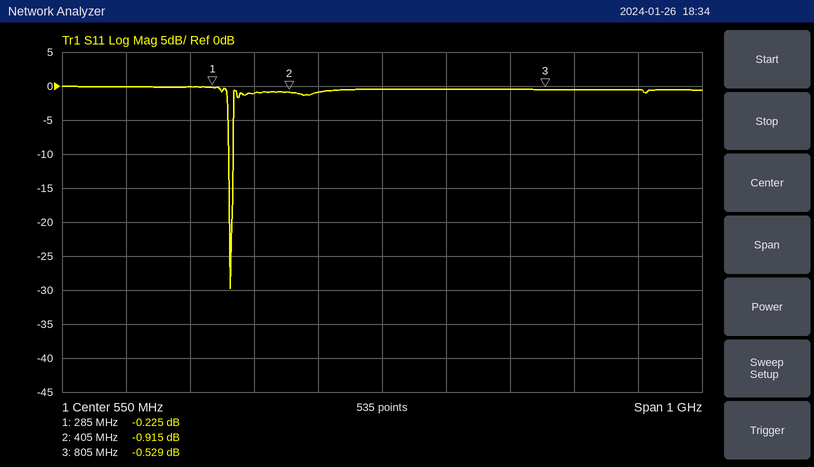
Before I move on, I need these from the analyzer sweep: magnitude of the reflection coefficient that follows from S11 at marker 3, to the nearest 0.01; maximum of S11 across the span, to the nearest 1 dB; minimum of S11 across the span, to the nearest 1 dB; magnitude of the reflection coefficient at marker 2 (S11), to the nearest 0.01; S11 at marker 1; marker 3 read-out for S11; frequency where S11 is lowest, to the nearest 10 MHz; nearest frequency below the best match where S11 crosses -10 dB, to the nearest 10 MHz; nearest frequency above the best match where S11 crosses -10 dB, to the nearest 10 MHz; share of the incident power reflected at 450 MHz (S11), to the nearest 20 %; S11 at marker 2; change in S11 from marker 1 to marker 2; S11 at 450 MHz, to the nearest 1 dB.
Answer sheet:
0.94
0 dB
-30 dB
0.90
-0.225 dB
-0.529 dB
310 MHz
310 MHz
320 MHz
80 %
-0.915 dB
-0.690 dB
-1 dB
